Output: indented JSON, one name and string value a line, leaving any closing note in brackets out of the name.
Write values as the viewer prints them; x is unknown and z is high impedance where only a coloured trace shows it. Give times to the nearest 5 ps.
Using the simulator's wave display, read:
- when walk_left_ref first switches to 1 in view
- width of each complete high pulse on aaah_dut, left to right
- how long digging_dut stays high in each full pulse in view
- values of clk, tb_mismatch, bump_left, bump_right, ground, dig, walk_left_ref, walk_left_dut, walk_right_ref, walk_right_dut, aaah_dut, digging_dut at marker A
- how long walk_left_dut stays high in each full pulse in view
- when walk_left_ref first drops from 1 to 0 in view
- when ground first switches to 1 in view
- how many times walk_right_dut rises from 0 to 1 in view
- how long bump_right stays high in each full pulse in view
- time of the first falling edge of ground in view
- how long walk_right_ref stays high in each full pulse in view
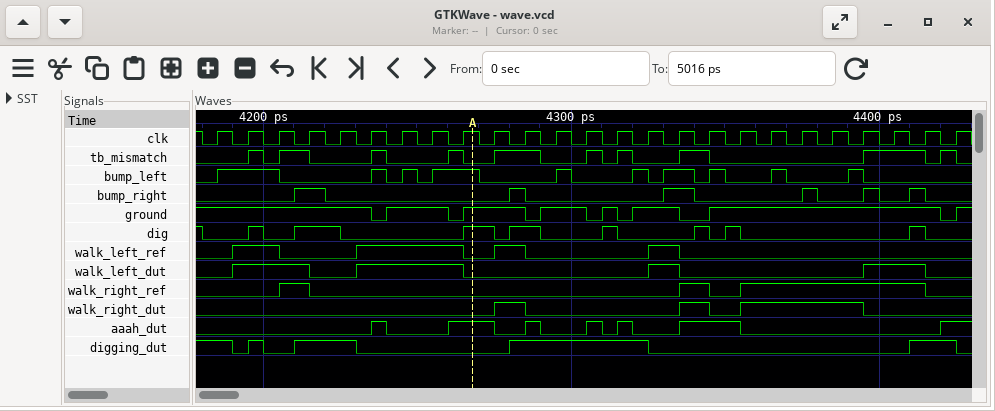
{
  "when walk_left_ref first switches to 1 in view": "4190 ps",
  "width of each complete high pulse on aaah_dut, left to right": "5 ps, 15 ps, 5 ps, 5 ps, 5 ps, 20 ps",
  "how long digging_dut stays high in each full pulse in view": "5 ps, 20 ps, 45 ps, 15 ps",
  "values of clk, tb_mismatch, bump_left, bump_right, ground, dig, walk_left_ref, walk_left_dut, walk_right_ref, walk_right_dut, aaah_dut, digging_dut at marker A": "clk=1, tb_mismatch=0, bump_left=1, bump_right=0, ground=1, dig=1, walk_left_ref=0, walk_left_dut=0, walk_right_ref=0, walk_right_dut=0, aaah_dut=1, digging_dut=0",
  "how long walk_left_dut stays high in each full pulse in view": "25 ps, 35 ps, 10 ps, 20 ps",
  "when walk_left_ref first drops from 1 to 0 in view": "4205 ps",
  "when ground first switches to 1 in view": "4240 ps",
  "how many times walk_right_dut rises from 0 to 1 in view": "3",
  "how long bump_right stays high in each full pulse in view": "10 ps, 5 ps, 10 ps, 5 ps, 5 ps, 5 ps",
  "time of the first falling edge of ground in view": "4235 ps",
  "how long walk_right_ref stays high in each full pulse in view": "10 ps, 10 ps, 60 ps"
}
